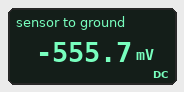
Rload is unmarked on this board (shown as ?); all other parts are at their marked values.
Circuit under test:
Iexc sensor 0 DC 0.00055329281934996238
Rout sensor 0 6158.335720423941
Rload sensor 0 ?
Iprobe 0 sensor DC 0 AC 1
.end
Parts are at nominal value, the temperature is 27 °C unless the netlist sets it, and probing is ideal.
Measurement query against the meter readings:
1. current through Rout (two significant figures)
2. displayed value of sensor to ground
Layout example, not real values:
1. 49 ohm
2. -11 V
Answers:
1. 90 µA
2. -555.7 mV
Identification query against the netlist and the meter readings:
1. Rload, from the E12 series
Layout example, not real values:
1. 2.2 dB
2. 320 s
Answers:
1. 1.2 kΩ
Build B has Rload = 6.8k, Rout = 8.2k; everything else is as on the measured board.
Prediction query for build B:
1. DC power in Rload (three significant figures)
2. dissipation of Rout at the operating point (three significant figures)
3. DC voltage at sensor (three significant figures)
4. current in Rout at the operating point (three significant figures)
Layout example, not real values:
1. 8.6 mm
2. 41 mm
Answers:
1. 622 µW
2. 516 µW
3. -2.06 V
4. 251 µA
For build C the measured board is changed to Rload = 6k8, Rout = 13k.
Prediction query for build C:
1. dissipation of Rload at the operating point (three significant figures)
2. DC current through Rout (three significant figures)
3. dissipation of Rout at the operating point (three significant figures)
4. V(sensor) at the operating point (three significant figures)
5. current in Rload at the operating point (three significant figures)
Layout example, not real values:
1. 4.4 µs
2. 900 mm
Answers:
1. 897 µW
2. 190 µA
3. 469 µW
4. -2.47 V
5. 363 µA
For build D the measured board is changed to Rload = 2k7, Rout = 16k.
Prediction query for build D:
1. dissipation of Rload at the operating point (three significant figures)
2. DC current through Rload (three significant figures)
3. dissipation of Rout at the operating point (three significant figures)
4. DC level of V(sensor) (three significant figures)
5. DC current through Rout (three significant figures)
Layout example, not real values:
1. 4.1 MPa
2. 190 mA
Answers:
1. 605 µW
2. 473 µA
3. 102 µW
4. -1.28 V
5. 79.9 µA
